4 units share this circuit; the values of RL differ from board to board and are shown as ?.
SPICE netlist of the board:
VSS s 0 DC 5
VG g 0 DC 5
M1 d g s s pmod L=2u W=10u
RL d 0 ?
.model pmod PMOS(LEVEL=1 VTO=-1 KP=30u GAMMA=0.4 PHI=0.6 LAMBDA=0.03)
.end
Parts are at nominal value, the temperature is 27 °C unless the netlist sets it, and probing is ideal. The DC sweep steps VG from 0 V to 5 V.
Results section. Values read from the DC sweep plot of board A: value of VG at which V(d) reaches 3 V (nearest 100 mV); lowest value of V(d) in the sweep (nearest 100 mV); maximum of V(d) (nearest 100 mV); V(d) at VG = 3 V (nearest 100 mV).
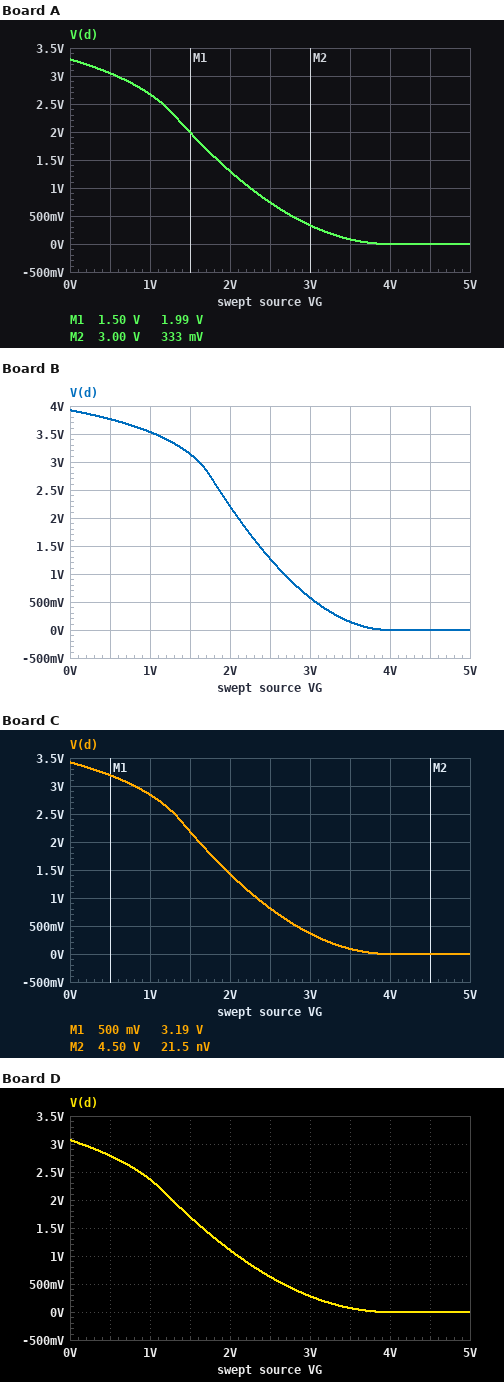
600 mV
0 V
3.3 V
300 mV
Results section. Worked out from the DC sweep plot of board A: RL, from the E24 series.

3.9 kΩ
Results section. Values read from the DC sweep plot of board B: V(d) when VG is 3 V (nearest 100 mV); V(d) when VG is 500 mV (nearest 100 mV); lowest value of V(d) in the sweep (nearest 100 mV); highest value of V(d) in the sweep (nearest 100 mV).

600 mV
3.8 V
0 V
3.9 V
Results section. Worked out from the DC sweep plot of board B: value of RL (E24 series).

6.8 kΩ
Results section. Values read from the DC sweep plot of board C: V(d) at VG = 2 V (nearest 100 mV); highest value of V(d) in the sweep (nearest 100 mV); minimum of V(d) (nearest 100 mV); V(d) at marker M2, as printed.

1.4 V
3.4 V
0 V
21.5 nV
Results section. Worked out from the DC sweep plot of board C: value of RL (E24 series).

4.3 kΩ
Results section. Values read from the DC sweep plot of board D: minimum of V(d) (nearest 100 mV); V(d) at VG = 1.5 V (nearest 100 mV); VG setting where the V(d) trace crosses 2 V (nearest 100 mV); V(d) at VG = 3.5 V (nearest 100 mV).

0 V
1.7 V
1.3 V
100 mV
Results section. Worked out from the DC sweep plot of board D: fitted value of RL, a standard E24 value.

3.3 kΩ
